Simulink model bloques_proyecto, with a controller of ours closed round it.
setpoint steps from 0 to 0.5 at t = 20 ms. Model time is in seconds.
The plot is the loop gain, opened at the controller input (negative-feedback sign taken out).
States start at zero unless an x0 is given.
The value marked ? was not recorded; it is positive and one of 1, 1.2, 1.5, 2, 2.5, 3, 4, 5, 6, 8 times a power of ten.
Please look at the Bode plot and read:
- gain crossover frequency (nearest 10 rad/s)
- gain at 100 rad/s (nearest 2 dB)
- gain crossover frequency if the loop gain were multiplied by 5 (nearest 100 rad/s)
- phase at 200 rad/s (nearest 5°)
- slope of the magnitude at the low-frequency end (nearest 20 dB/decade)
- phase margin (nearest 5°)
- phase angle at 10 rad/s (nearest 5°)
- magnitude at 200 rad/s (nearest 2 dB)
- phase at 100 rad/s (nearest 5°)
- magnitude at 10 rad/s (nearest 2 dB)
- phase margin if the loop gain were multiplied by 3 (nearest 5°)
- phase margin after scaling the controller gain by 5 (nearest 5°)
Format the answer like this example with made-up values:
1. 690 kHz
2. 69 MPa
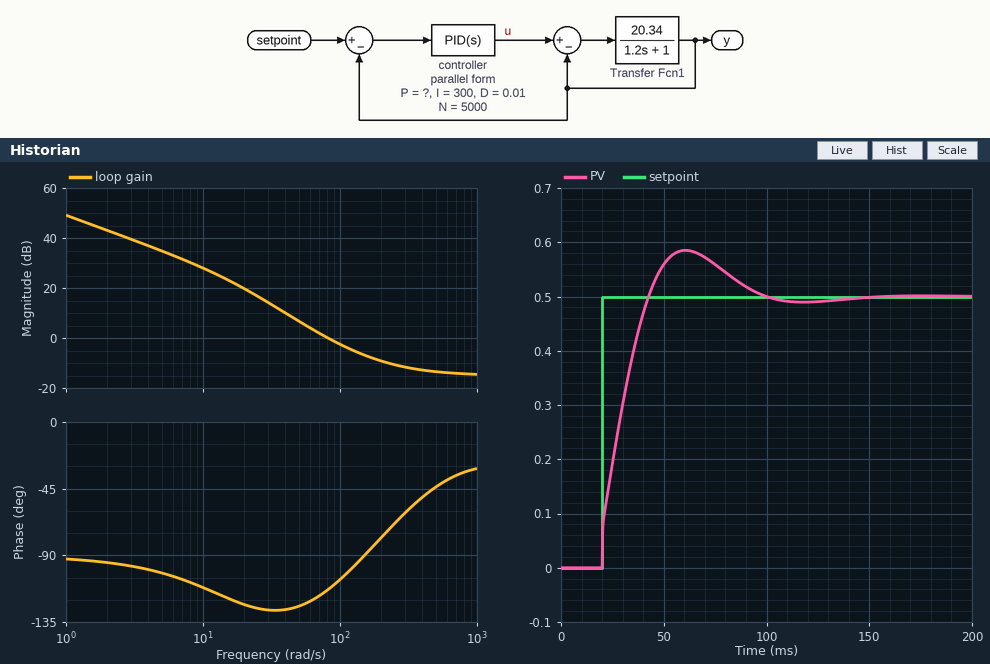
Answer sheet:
1. 80 rad/s
2. -2 dB
3. 600 rad/s
4. -80°
5. -20 dB/decade
6. 65°
7. -110°
8. -10 dB
9. -105°
10. 28 dB
11. 105°
12. 140°
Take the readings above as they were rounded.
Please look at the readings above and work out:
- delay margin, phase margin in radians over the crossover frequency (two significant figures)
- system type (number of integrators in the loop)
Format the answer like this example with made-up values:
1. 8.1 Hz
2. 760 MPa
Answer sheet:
1. 0.014 s
2. 1
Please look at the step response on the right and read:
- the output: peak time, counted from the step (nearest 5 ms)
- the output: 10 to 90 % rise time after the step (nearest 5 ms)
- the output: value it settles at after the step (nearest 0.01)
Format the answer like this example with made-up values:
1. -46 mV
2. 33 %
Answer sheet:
1. 40 ms
2. 20 ms
3. 0.50
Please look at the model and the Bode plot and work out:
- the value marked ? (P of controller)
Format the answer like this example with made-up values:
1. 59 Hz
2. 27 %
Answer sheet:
1. 4
